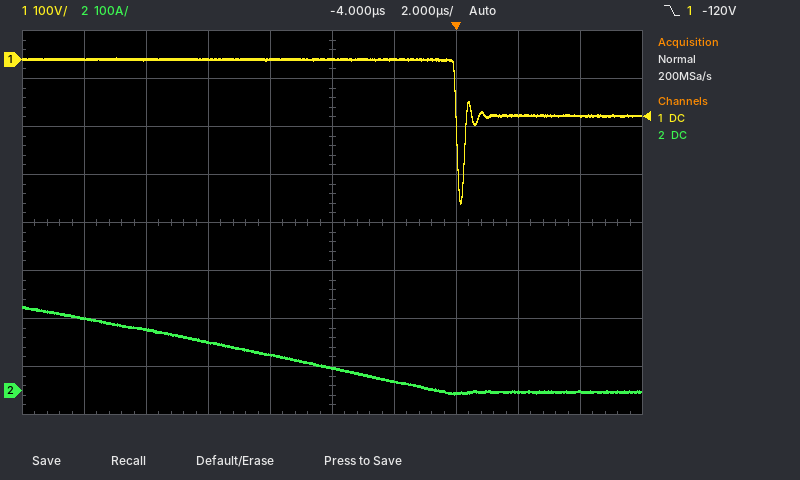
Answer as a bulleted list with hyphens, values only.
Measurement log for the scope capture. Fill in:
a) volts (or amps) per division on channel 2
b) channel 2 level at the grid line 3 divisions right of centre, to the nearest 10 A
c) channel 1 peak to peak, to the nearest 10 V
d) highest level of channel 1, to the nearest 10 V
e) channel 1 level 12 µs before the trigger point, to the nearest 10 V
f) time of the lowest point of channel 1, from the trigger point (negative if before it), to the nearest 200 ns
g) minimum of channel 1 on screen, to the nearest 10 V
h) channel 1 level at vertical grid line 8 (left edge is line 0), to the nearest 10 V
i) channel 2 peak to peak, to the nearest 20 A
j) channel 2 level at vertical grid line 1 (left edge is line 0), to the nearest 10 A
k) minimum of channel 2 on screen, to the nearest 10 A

- 100 A
- 0 A
- 300 V
- 0 V
- 0 V
- +200 ns
- -300 V
- -120 V
- 180 A
- 150 A
- -10 A
